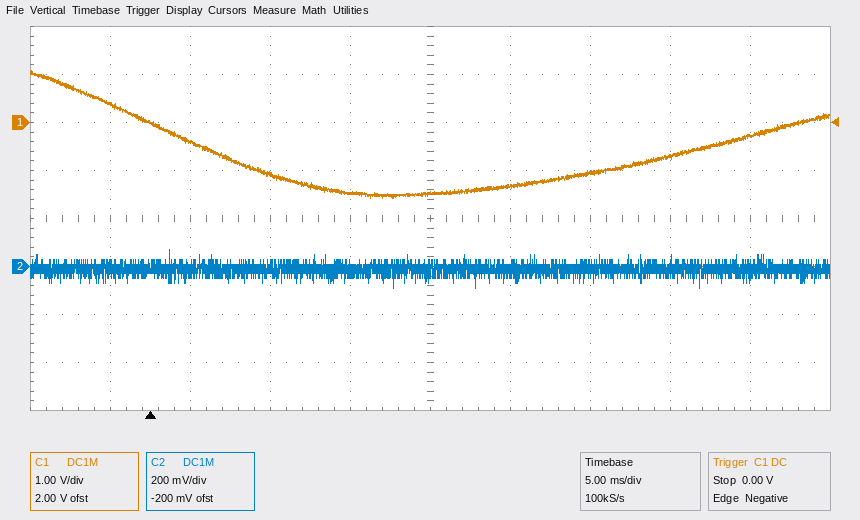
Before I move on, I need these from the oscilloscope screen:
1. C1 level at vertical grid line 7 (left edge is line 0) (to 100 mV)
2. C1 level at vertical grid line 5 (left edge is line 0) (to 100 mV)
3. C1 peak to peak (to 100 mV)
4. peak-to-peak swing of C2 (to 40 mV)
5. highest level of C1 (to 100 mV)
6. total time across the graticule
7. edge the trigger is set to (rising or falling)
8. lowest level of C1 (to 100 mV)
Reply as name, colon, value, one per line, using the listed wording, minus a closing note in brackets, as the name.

C1 level at vertical grid line 7 (left edge is line 0): -1.1 V
C1 level at vertical grid line 5 (left edge is line 0): -1.5 V
C1 peak to peak: 2.7 V
peak-to-peak swing of C2: 160 mV
highest level of C1: 1.1 V
total time across the graticule: 50 ms
edge the trigger is set to: falling
lowest level of C1: -1.6 V
